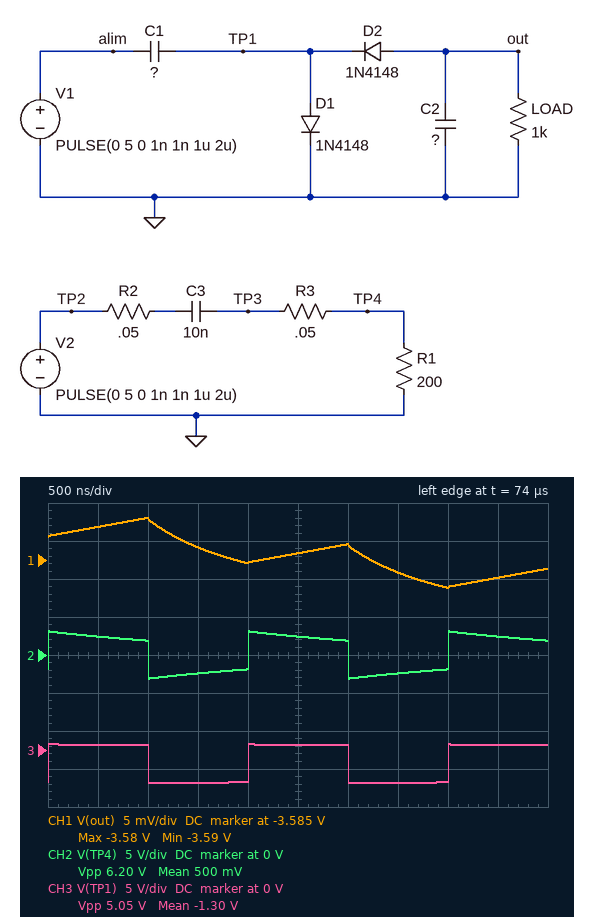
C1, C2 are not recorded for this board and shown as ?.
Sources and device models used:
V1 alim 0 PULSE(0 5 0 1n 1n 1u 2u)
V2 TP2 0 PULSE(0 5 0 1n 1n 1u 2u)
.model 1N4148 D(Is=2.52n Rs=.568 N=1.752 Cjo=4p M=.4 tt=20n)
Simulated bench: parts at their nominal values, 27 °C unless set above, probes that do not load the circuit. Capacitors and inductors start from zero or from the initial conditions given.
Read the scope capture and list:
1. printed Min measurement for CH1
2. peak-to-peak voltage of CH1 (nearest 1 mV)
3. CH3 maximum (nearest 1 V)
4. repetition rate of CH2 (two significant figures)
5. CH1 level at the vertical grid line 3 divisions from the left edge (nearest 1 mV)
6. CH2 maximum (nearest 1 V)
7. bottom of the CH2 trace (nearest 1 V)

-3.59 V
9 mV
1 V
500 kHz
-3.583 V
3 V
-3 V
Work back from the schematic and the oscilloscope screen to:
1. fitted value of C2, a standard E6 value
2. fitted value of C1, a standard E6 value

1.5 µF
330 nF
